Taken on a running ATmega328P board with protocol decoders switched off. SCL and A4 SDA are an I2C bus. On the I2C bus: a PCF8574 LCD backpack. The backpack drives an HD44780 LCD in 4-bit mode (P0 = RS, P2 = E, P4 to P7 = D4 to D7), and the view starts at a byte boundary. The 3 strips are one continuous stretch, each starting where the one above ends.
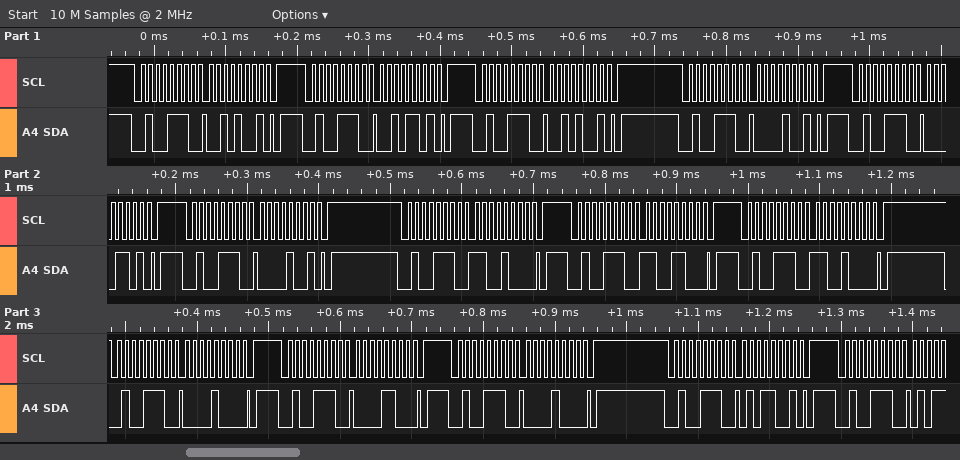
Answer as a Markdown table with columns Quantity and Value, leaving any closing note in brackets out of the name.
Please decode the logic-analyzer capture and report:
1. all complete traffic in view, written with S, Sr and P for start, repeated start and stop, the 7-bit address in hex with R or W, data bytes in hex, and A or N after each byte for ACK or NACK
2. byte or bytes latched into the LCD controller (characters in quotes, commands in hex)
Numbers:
| Quantity | Value |
|---|---|
| all complete traffic in view, written with S, Sr and P for start, repeated start and stop, the 7-bit address in hex with R or W, data bytes in hex, and A or N after each byte for ACK or NACK | S 27W A 29 A P S 27W A 2D A P S 27W A 29 A P S 27W A 09 A P S 27W A 0D A P S 27W A 09 A P S 27W A C8 A P S 27W A CC A P S 27W A C8 A P S 27W A 08 A P S 27W A 0C A P S 27W A 08 A P S 27W A 59 A P S 27W A |
| byte or bytes latched into the LCD controller | ' ' 0xC0 |
